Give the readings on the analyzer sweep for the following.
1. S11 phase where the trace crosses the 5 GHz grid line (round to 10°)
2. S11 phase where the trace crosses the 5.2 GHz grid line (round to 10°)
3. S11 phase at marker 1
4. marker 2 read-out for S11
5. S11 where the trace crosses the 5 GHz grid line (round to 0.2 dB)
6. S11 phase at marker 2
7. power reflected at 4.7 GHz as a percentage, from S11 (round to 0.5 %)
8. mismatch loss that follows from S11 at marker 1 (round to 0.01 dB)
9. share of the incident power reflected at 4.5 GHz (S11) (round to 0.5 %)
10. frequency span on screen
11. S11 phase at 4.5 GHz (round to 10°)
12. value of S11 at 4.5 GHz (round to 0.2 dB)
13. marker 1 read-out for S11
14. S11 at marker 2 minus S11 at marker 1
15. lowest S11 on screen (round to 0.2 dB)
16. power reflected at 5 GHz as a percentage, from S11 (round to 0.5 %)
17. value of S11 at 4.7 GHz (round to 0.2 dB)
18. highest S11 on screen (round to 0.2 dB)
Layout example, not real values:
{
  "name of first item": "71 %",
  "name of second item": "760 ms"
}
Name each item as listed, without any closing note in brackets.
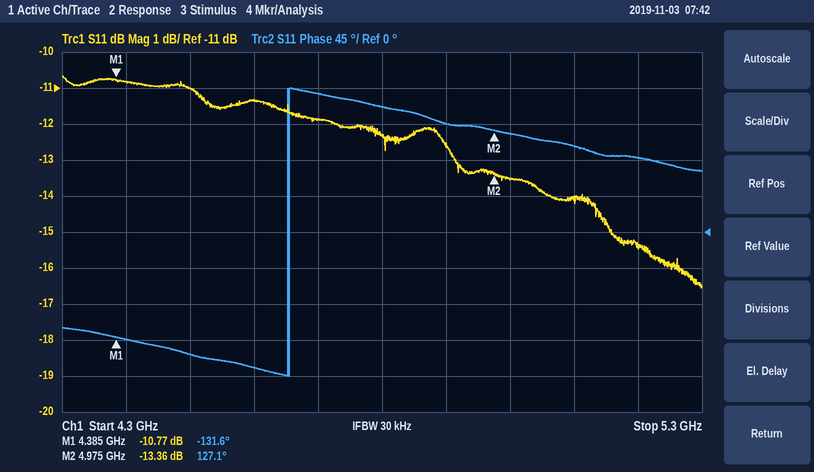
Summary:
{
  "S11 phase where the trace crosses the 5 GHz grid line": "120°",
  "S11 phase where the trace crosses the 5.2 GHz grid line": "90°",
  "S11 phase at marker 1": "-131.6°",
  "marker 2 read-out for S11": "-13.36 dB",
  "S11 where the trace crosses the 5 GHz grid line": "-13.6 dB",
  "S11 phase at marker 2": "127.1°",
  "power reflected at 4.7 GHz as a percentage, from S11": "6.5 %",
  "mismatch loss that follows from S11 at marker 1": "0.38 dB",
  "share of the incident power reflected at 4.5 GHz (S11)": "8.0 %",
  "frequency span on screen": "1 GHz",
  "S11 phase at 4.5 GHz": "-150°",
  "value of S11 at 4.5 GHz": "-11.0 dB",
  "marker 1 read-out for S11": "-10.77 dB",
  "S11 at marker 2 minus S11 at marker 1": "-2.59 dB",
  "lowest S11 on screen": "-16.6 dB",
  "power reflected at 5 GHz as a percentage, from S11": "4.5 %",
  "value of S11 at 4.7 GHz": "-11.8 dB",
  "highest S11 on screen": "-10.6 dB"
}
